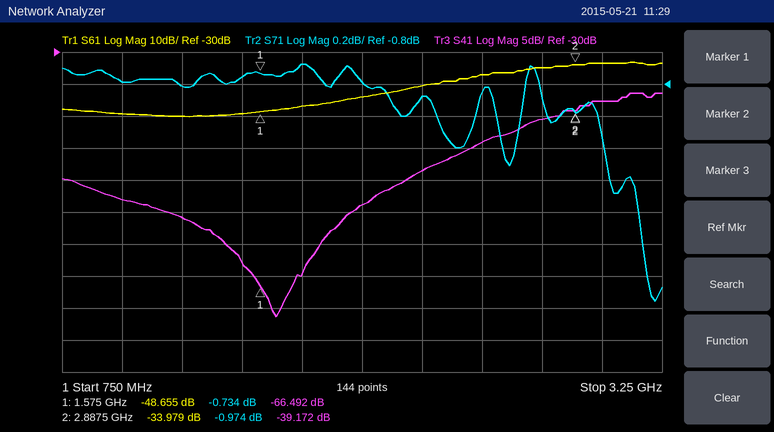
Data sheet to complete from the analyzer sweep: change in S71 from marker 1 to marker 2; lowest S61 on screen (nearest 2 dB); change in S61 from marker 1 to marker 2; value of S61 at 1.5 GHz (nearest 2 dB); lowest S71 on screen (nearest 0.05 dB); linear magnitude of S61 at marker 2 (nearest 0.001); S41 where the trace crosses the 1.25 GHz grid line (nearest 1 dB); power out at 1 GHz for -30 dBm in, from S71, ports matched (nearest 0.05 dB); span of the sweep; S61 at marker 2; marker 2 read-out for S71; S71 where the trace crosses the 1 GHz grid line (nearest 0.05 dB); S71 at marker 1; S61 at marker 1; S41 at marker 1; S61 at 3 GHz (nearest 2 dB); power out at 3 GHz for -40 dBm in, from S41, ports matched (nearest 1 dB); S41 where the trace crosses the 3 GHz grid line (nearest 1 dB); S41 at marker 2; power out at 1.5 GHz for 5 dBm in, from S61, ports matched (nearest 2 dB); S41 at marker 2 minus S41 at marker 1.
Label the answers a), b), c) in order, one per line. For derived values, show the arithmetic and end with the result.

a) -0.974 − (-0.734) = -0.240 dB
b) -50 dB
c) -33.979 − (-48.655) = 14.676 dB
d) -50 dB
e) -2.15 dB
f) 10^(-33.979/20) ≈ 0.020
g) -56 dB
h) -30 dBm + (-0.80 dB) = -30.80 dBm
i) 2.5 GHz
j) -33.979 dB
k) -0.974 dB
l) -0.80 dB
m) -0.734 dB
n) -48.655 dB
o) -66.492 dB
p) -34 dB
q) -40 dBm + (-38 dB) = -78 dBm
r) -38 dB
s) -39.172 dB
t) 5 dBm + (-50 dB) = -44 dBm
u) -39.172 − (-66.492) = 27.320 dB
